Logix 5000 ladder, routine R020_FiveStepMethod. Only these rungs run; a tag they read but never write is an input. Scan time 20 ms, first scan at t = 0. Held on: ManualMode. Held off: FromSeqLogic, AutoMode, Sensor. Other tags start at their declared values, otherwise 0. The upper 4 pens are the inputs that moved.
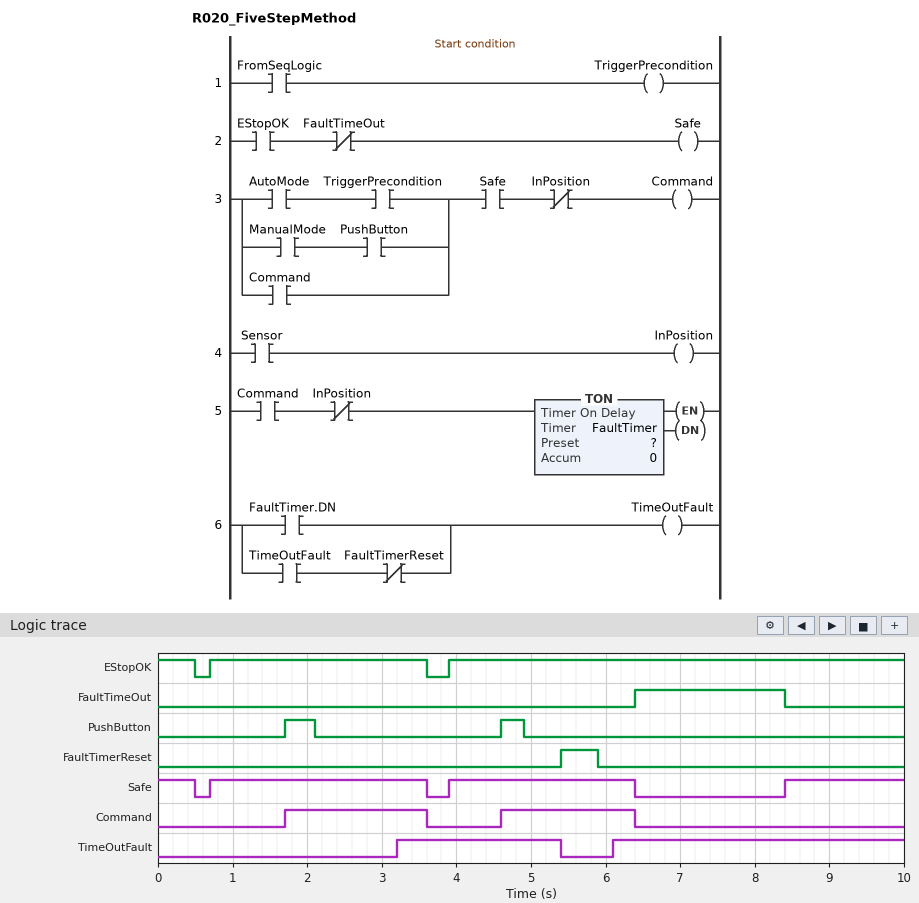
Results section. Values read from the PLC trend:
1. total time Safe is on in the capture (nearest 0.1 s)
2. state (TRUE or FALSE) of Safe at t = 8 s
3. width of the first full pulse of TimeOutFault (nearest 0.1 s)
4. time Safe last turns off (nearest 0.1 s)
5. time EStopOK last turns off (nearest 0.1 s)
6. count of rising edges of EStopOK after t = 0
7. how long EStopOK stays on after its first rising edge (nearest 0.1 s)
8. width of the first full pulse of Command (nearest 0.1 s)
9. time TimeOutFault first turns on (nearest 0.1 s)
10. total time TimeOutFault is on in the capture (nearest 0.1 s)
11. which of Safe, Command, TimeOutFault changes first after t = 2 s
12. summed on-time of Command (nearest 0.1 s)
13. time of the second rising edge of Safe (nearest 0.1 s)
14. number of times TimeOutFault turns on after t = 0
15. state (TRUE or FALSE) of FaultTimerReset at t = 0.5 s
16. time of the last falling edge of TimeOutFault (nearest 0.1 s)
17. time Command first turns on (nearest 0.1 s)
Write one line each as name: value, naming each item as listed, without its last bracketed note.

total time Safe is on in the capture: 7.5 s
state (TRUE or FALSE) of Safe at t = 8 s: FALSE
width of the first full pulse of TimeOutFault: 2.2 s
time Safe last turns off: 6.4 s
time EStopOK last turns off: 3.6 s
count of rising edges of EStopOK after t = 0: 2
how long EStopOK stays on after its first rising edge: 2.9 s
width of the first full pulse of Command: 1.9 s
time TimeOutFault first turns on: 3.2 s
total time TimeOutFault is on in the capture: 6.1 s
which of Safe, Command, TimeOutFault changes first after t = 2 s: TimeOutFault
summed on-time of Command: 3.7 s
time of the second rising edge of Safe: 3.9 s
number of times TimeOutFault turns on after t = 0: 2
state (TRUE or FALSE) of FaultTimerReset at t = 0.5 s: FALSE
time of the last falling edge of TimeOutFault: 5.4 s
time Command first turns on: 1.7 s
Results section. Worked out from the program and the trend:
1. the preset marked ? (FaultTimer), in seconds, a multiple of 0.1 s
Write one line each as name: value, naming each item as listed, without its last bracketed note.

the preset marked ? (FaultTimer), in seconds, a multiple of 0.1 s: 1.5 s
